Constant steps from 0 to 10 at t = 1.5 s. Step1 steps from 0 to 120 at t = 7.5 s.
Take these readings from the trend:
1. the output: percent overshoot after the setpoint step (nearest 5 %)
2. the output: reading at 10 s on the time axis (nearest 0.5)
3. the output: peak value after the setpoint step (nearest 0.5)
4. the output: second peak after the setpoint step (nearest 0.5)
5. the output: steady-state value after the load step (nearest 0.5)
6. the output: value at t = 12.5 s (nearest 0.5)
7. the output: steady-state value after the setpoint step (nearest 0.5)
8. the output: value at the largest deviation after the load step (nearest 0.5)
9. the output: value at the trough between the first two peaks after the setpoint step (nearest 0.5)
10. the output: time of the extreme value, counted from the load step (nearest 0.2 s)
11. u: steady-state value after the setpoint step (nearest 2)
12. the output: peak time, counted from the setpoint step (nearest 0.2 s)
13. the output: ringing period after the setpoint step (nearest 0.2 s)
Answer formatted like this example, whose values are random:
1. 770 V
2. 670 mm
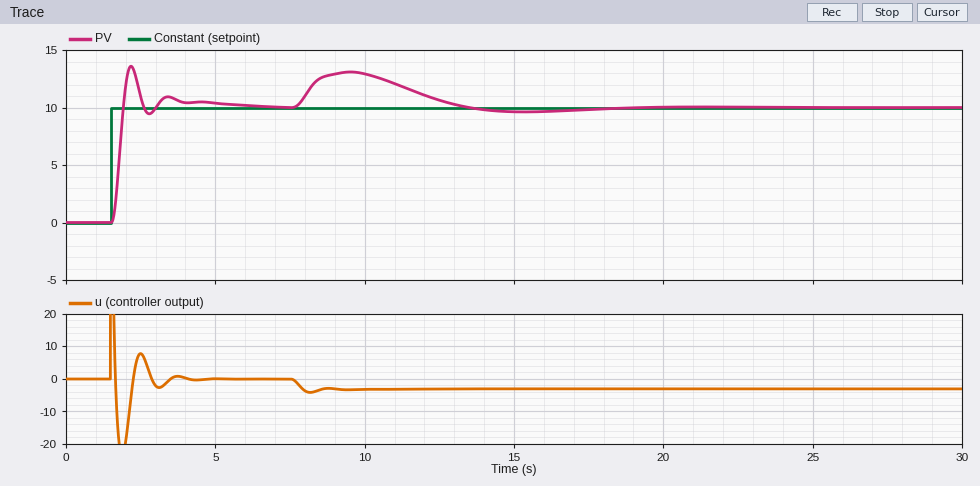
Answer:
1. 35 %
2. 13.0
3. 13.5
4. 11.0
5. 10.0
6. 10.5
7. 10.0
8. 13.0
9. 9.5
10. 2.0 s
11. 0
12. 0.6 s
13. 1.2 s
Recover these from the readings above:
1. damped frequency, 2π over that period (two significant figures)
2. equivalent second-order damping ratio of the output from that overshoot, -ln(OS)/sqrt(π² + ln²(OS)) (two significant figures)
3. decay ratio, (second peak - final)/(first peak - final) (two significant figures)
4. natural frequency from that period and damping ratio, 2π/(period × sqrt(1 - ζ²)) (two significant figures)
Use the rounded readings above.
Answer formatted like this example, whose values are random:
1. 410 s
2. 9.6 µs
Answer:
1. 5.2 rad/s
2. 0.32
3. 0.29
4. 5.5 rad/s
